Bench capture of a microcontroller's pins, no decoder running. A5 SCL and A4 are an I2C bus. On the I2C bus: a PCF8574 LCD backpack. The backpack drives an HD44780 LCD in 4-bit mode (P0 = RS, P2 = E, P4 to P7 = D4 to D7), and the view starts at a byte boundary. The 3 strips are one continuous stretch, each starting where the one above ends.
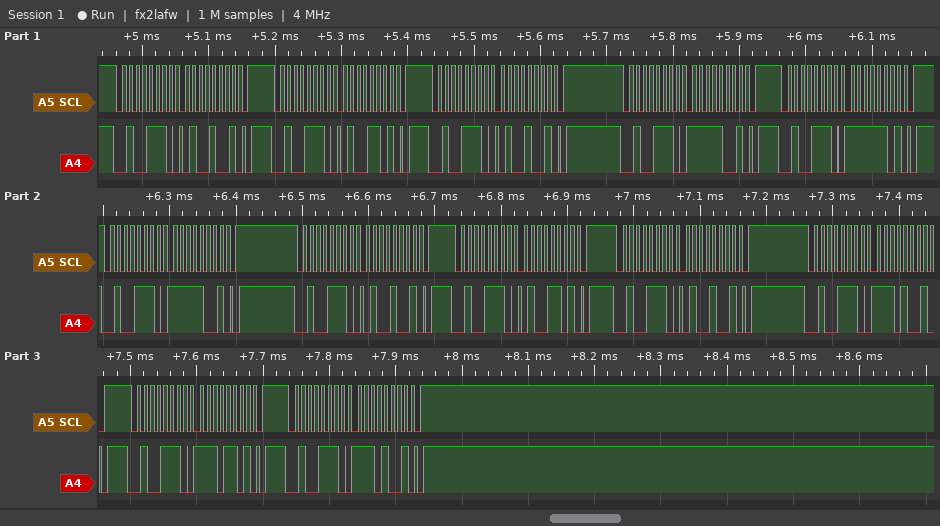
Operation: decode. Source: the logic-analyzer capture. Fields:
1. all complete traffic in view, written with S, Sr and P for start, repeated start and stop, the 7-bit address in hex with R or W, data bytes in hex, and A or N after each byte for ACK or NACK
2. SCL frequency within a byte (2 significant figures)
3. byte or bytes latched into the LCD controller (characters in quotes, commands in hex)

S 27W A 49 A P S 27W A 4D A P S 27W A 49 A P S 27W A F9 A P S 27W A FD A P S 27W A F9 A P S 27W A 49 A P S 27W A 4D A P S 27W A 49 A P S 27W A E9 A P S 27W A ED A P S 27W A E9 A P
100 kHz
'O' 'N'
